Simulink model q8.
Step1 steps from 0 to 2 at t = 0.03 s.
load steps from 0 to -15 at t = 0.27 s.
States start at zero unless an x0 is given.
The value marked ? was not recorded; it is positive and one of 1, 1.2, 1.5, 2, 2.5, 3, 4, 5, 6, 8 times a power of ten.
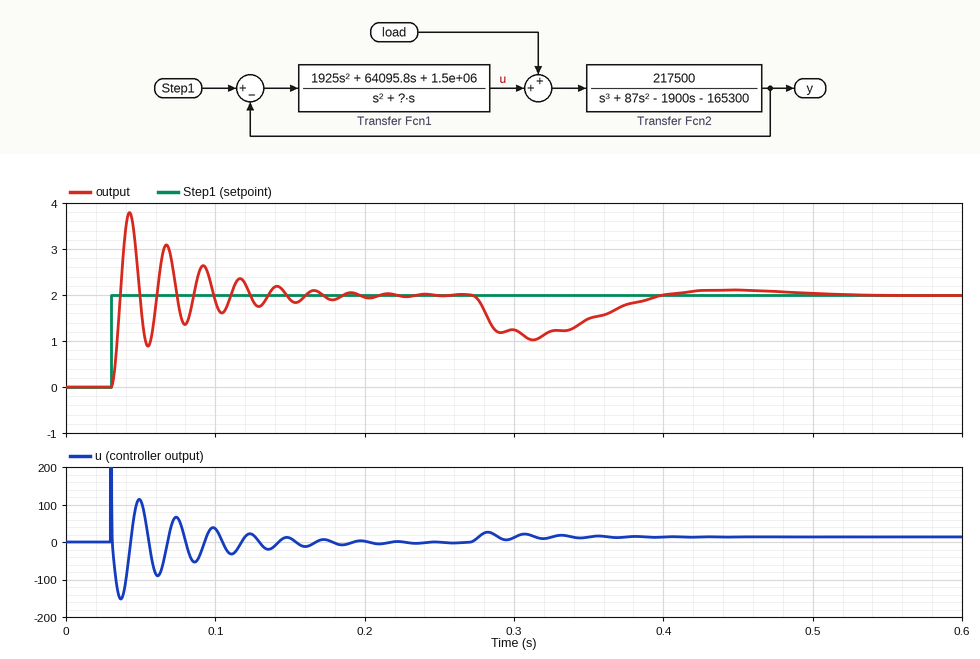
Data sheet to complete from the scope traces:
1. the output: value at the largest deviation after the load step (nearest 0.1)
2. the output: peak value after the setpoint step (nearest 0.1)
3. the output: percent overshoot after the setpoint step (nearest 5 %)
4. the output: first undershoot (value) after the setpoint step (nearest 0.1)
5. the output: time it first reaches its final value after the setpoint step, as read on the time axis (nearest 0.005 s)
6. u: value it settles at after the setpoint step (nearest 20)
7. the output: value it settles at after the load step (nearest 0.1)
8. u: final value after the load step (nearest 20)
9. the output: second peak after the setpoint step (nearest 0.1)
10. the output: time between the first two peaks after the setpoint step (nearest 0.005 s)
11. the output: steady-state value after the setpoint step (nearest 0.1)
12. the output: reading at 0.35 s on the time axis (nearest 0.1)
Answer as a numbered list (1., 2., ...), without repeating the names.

1. 1.0
2. 3.8
3. 90 %
4. 0.9
5. 0.035 s
6. 0
7. 2.0
8. 20
9. 3.1
10. 0.025 s
11. 2.0
12. 1.5
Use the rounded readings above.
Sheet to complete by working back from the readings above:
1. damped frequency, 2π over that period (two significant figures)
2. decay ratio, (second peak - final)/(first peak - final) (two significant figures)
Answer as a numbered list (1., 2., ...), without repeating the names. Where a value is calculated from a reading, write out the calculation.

1. 2π / 0.025 = 250 rad/s
2. (3.1 - 2) / (3.8 - 2) = 0.61
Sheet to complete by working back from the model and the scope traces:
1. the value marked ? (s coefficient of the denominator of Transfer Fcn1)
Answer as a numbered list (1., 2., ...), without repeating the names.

1. 6000
